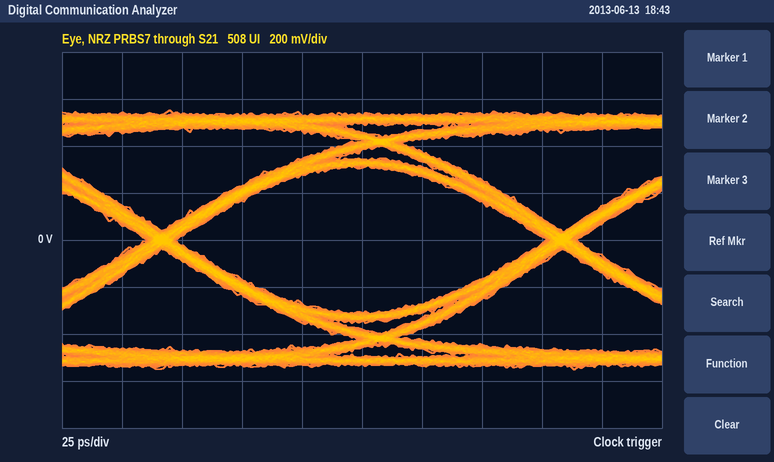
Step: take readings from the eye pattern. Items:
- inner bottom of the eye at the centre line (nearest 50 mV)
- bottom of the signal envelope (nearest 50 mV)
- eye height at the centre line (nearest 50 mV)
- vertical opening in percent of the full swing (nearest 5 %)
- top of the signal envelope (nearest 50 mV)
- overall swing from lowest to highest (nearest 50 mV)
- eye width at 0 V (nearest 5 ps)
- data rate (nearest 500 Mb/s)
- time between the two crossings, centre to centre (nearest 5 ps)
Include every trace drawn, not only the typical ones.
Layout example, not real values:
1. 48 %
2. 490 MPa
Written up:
1. -300 mV
2. -550 mV
3. 600 mV
4. 55 %
5. 550 mV
6. 1.10 V
7. 155 ps
8. 6.0 Gb/s
9. 165 ps
